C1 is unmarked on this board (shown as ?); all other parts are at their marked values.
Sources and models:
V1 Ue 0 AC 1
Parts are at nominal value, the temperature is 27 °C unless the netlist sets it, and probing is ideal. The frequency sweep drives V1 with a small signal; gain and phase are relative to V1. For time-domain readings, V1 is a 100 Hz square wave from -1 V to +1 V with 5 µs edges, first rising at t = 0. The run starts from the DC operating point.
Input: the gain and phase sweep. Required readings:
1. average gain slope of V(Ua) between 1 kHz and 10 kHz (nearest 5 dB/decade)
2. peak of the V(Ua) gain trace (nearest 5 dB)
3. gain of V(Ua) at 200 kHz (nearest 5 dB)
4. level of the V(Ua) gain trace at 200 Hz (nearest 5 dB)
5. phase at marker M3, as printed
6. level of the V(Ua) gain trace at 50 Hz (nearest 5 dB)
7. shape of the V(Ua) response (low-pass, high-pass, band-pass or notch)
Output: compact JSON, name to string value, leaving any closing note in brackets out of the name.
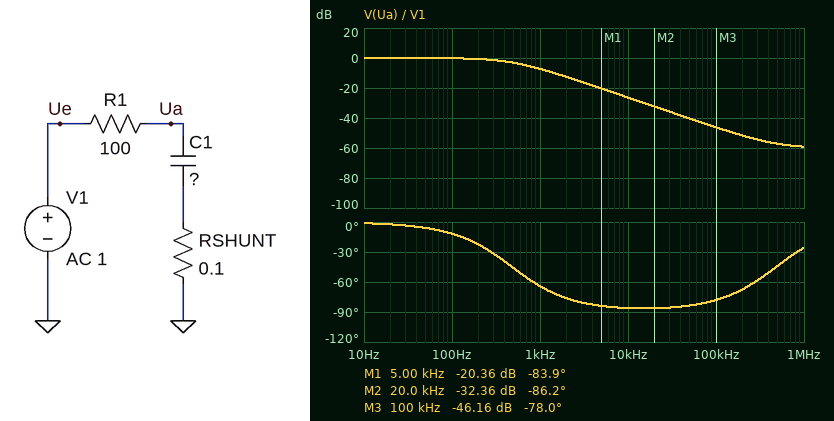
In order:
{"average gain slope of V(Ua) between 1 kHz and 10 kHz": "-20 dB/decade", "peak of the V(Ua) gain trace": "0 dB", "gain of V(Ua) at 200 kHz": "-50 dB", "level of the V(Ua) gain trace at 200 Hz": "0 dB", "phase at marker M3, as printed": "-78.0 deg", "level of the V(Ua) gain trace at 50 Hz": "0 dB", "shape of the V(Ua) response": "low-pass"}
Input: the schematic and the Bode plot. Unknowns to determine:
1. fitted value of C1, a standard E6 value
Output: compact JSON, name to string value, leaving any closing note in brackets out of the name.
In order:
{"fitted value of C1, a standard E6 value": "3.3 µF"}
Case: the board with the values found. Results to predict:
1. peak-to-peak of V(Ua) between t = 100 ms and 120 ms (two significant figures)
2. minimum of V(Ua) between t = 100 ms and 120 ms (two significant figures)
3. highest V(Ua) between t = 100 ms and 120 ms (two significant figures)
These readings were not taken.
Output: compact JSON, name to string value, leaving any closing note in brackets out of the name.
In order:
{"peak-to-peak of V(Ua) between t = 100 ms and 120 ms": "2.0 V", "minimum of V(Ua) between t = 100 ms and 120 ms": "-1.0 V", "highest V(Ua) between t = 100 ms and 120 ms": "1.0 V"}
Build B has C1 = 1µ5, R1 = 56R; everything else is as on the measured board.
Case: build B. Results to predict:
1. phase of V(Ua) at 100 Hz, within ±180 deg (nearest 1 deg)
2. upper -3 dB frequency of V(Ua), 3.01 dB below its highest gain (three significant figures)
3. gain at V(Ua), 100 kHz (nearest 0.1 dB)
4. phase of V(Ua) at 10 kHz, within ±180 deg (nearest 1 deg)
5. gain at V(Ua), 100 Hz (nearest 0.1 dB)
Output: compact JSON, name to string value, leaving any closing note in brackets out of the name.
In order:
{"phase of V(Ua) at 100 Hz, within ±180 deg": "-3 deg", "upper -3 dB frequency of V(Ua), 3.01 dB below its highest gain": "1.89 kHz", "gain at V(Ua), 100 kHz": "-34.4 dB", "phase of V(Ua) at 10 kHz, within ±180 deg": "-79 deg", "gain at V(Ua), 100 Hz": "0 dB"}
